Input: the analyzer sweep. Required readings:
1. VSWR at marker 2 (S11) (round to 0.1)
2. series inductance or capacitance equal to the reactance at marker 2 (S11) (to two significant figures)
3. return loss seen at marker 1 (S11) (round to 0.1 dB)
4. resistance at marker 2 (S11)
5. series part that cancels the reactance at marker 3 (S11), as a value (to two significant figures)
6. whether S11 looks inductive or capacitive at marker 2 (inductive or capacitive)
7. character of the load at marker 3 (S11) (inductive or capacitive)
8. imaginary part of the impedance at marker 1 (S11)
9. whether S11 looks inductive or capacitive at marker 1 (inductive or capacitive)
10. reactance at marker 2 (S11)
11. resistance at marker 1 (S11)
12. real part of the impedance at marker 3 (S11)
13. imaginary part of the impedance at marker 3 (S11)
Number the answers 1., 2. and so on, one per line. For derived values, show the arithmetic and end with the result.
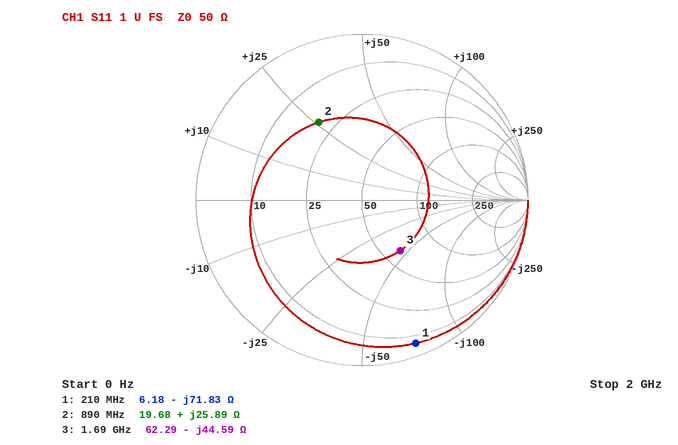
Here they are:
1. 3.3
2. L = 25.89 Ω/(2π × 890 MHz) ≈ 4.6 nH
3. 0.7 dB
4. 19.68 Ω
5. L = 44.59 Ω/(2π × 1.69 GHz) ≈ 4.2 nH
6. inductive
7. capacitive
8. -71.83 Ω
9. capacitive
10. +25.89 Ω
11. 6.18 Ω
12. 62.29 Ω
13. -44.59 Ω
